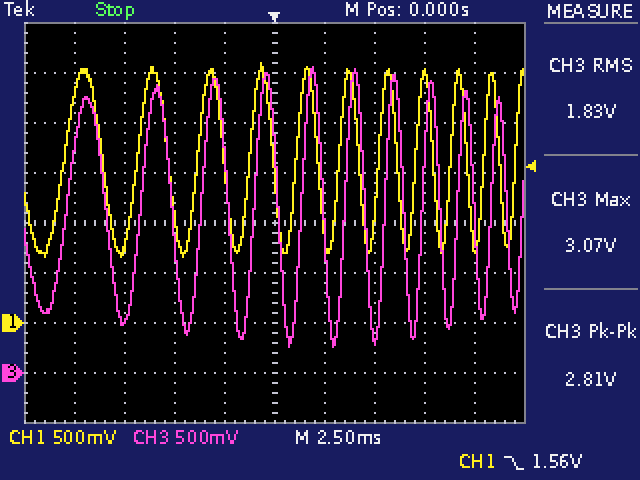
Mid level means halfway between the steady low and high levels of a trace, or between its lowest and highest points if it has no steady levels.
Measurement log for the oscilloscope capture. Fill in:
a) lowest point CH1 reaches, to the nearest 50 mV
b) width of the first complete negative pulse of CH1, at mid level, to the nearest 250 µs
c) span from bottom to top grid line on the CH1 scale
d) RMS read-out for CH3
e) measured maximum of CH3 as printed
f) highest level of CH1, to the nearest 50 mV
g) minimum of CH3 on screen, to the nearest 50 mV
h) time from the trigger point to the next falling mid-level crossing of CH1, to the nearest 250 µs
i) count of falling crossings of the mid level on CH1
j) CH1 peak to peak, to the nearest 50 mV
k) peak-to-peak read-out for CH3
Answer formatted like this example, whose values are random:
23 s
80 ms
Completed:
650 mV
1.75 ms
4 V
1.83 V
3.07 V
2.60 V
250 mV
2.25 ms
10
1.95 V
2.81 V
